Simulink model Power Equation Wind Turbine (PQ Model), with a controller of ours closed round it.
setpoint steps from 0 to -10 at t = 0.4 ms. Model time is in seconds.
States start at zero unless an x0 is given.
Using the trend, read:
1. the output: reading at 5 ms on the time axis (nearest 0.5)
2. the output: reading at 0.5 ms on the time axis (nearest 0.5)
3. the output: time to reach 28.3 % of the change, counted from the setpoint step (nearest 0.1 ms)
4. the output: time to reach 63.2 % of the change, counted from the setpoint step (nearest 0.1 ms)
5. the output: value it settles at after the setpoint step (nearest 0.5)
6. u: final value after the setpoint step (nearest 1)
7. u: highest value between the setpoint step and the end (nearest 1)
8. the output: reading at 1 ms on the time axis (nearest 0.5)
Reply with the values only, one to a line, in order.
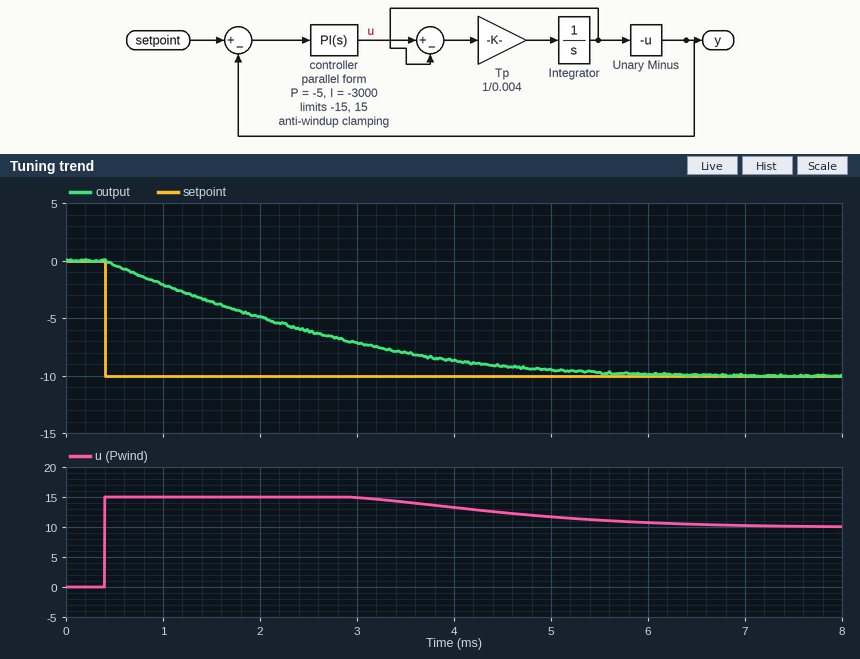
-9.5
-0.5
0.8 ms
2.2 ms
-10.0
10
15
-2.0
